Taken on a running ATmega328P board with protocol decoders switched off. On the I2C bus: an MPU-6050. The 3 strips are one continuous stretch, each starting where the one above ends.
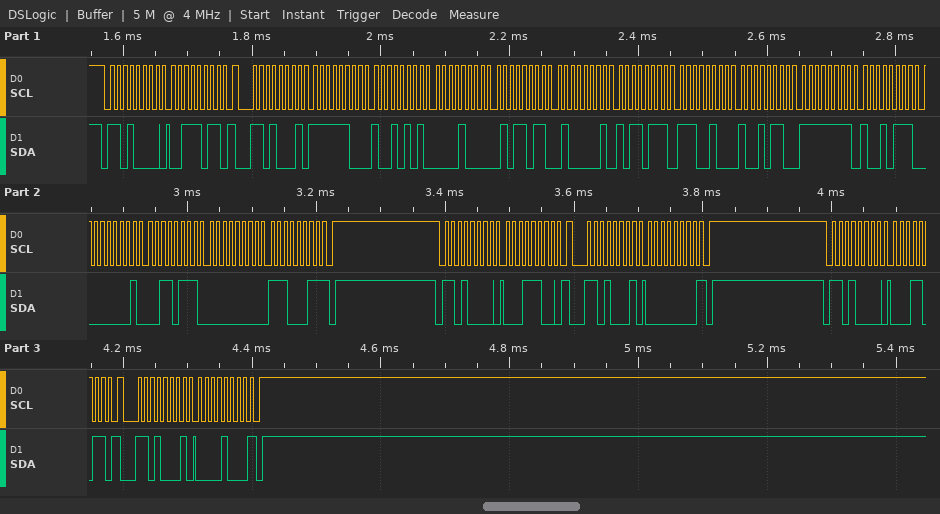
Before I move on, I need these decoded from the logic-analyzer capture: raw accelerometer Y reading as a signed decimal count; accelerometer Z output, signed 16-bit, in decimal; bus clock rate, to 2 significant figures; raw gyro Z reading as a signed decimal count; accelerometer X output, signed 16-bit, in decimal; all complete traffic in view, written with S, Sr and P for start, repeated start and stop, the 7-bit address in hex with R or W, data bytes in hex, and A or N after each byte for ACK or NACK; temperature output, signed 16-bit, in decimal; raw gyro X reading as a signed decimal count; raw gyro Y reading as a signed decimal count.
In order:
2139
16823
100 kHz
227
-875
S 68W A 3B A Sr 68R A FC A 95 A 08 A 5B A 41 A B7 A E4 A 96 A FF A 97 A 01 A 37 A 00 A E3 N P S 68W A 1C A Sr 68R A 00 N P S 68W A 1B A Sr 68R A 08 N P
-7018
-105
311
